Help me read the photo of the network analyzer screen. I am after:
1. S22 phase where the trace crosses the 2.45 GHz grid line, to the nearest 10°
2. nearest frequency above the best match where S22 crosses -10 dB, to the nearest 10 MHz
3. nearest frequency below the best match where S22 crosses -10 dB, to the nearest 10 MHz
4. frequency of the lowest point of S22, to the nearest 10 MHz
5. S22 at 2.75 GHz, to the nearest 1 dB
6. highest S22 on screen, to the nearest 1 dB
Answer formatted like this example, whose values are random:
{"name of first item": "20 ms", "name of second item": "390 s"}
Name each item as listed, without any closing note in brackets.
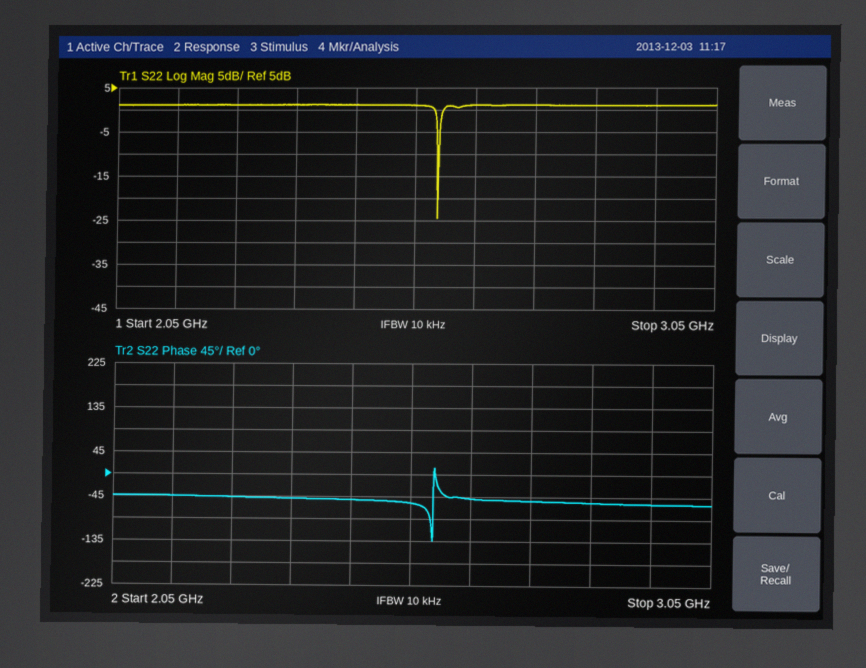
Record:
{"S22 phase where the trace crosses the 2.45 GHz grid line, to the nearest 10°": "-50°", "nearest frequency above the best match where S22 crosses -10 dB, to the nearest 10 MHz": "2.59 GHz", "nearest frequency below the best match where S22 crosses -10 dB, to the nearest 10 MHz": "2.59 GHz", "frequency of the lowest point of S22, to the nearest 10 MHz": "2.59 GHz", "S22 at 2.75 GHz, to the nearest 1 dB": "1 dB", "highest S22 on screen, to the nearest 1 dB": "1 dB"}
